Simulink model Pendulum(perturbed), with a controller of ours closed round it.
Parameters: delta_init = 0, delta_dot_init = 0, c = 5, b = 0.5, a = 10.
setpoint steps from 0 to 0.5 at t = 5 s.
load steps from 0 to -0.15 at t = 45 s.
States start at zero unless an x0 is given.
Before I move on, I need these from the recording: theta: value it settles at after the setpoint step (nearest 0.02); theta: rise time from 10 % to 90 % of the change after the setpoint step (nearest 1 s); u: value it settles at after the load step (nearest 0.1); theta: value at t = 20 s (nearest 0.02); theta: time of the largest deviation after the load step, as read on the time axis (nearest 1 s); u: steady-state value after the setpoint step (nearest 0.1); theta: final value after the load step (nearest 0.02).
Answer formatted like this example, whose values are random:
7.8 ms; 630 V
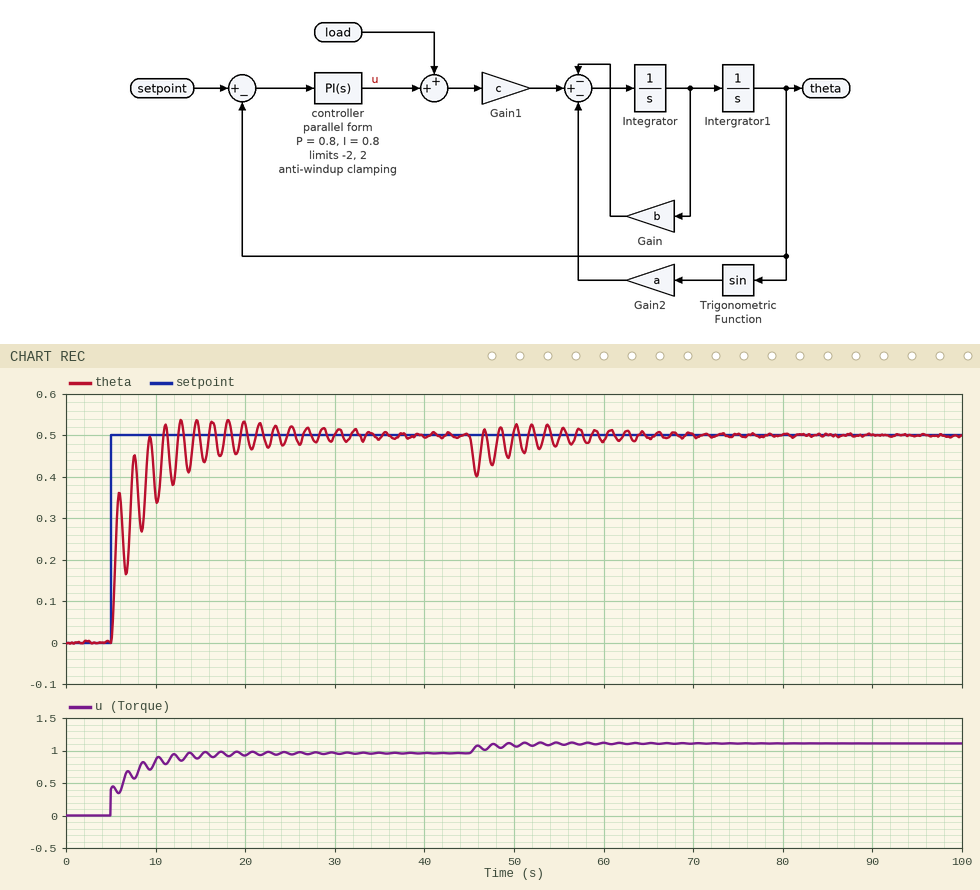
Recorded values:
0.50; 4 s; 1.1; 0.52; 46 s; 1.0; 0.50
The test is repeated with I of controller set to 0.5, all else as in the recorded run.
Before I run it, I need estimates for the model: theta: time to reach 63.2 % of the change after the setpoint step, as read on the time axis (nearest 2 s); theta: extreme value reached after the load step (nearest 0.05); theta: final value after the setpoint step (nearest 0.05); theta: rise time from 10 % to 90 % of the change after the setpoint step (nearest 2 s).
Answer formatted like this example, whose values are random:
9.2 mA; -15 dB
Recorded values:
6 s; 0.40; 0.50; 8 s
